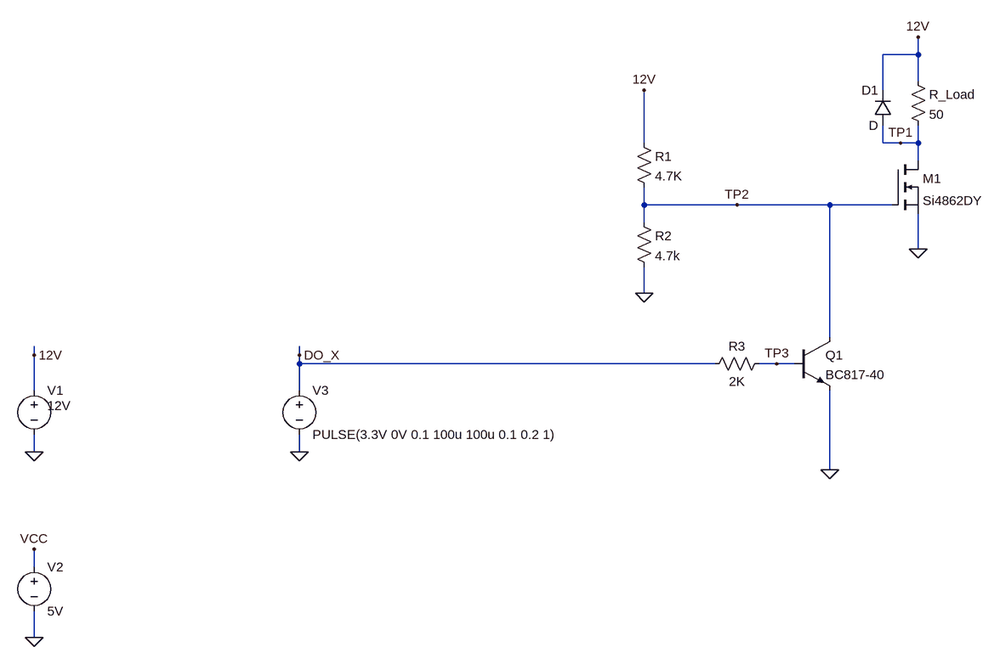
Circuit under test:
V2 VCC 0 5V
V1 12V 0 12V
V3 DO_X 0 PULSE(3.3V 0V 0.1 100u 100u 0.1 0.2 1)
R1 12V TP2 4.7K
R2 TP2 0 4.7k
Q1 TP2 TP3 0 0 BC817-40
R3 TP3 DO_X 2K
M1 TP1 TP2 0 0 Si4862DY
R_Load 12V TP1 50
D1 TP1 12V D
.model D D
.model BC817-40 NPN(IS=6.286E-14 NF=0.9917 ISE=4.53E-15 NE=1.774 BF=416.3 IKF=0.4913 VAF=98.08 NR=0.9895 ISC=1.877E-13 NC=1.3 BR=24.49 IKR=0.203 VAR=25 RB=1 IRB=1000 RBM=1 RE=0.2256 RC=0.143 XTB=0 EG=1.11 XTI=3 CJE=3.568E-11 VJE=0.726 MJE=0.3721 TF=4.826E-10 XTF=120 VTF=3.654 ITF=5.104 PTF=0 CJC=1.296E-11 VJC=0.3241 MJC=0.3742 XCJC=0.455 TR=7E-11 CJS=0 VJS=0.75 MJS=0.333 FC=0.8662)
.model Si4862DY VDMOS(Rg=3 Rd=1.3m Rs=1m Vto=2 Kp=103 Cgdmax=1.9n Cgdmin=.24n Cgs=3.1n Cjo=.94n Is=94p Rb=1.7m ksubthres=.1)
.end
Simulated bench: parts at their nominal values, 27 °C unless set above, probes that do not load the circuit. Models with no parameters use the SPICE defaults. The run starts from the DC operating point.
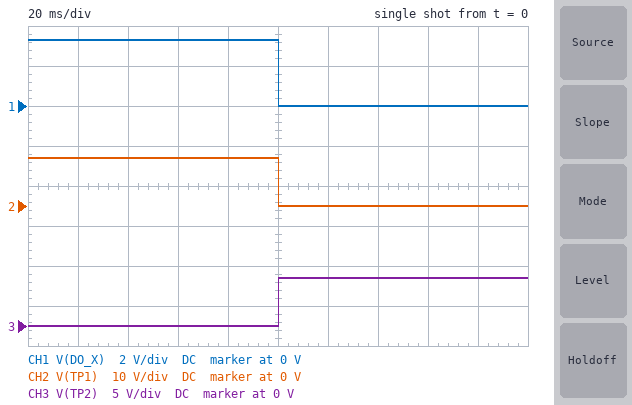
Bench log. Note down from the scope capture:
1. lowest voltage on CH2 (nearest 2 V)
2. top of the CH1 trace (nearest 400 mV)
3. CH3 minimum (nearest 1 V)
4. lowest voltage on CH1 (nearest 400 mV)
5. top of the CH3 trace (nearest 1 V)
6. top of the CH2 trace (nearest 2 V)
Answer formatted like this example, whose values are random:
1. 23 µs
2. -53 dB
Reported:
1. 0 V
2. 3.2 V
3. 0 V
4. 0 V
5. 6 V
6. 12 V
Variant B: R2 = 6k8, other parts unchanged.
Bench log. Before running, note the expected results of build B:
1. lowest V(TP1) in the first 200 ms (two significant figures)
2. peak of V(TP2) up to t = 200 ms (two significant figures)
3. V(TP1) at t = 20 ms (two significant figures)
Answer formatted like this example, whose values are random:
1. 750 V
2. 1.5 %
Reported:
1. 1.0 mV
2. 7.1 V
3. 12 V
